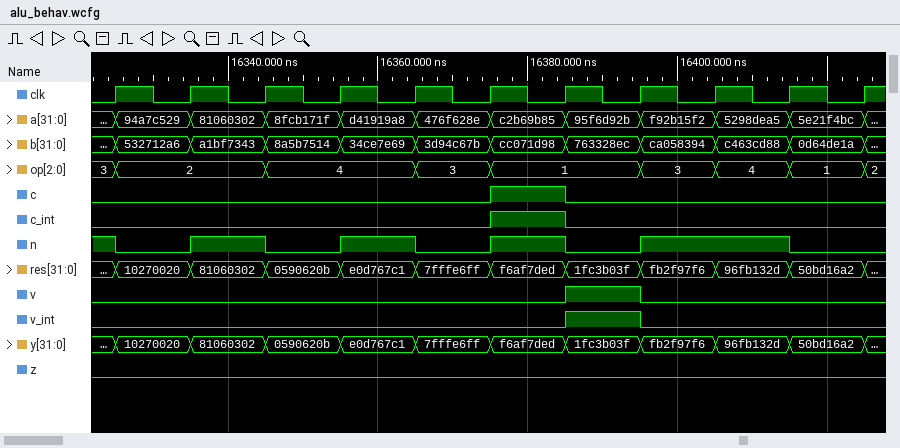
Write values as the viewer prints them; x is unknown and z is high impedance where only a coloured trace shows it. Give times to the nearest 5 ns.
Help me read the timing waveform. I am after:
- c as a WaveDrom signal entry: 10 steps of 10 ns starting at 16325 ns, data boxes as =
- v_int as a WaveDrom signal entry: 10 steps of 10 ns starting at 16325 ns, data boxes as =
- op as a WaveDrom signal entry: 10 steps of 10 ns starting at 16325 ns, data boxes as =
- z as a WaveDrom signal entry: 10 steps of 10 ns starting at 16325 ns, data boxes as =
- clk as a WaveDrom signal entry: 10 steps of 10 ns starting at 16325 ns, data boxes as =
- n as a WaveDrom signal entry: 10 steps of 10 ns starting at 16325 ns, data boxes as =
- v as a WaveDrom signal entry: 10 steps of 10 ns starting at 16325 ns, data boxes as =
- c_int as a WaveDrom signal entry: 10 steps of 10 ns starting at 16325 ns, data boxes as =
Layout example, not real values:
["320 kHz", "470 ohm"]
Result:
["{name: 'c', wave: '0....10...'}", "{name: 'v_int', wave: '0.....10..'}", "{name: 'op', wave: '=.=.==.===', data: '2 4 3 1 3 4 1'}", "{name: 'z', wave: '0.........'}", "{name: 'clk', wave: 'p.........'}", "{name: 'n', wave: '01010101.0'}", "{name: 'v', wave: '0.....10..'}", "{name: 'c_int', wave: '0....10...'}"]
